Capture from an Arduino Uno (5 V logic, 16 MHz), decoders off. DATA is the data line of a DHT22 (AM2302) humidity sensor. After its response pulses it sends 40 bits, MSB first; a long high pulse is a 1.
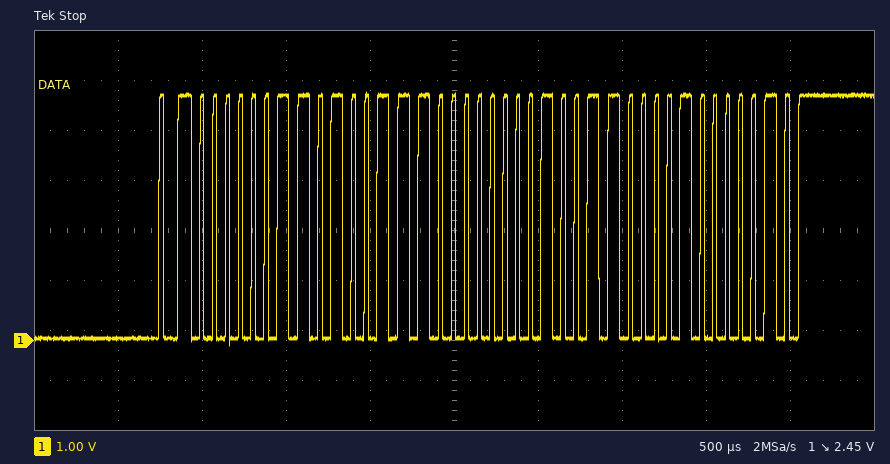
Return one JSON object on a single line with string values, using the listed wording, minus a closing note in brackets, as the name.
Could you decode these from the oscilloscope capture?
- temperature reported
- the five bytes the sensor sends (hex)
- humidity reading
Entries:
{"temperature reported": "30.4 °C", "the five bytes the sensor sends": "03 4E 01 30 82", "humidity reading": "84.6 %"}
